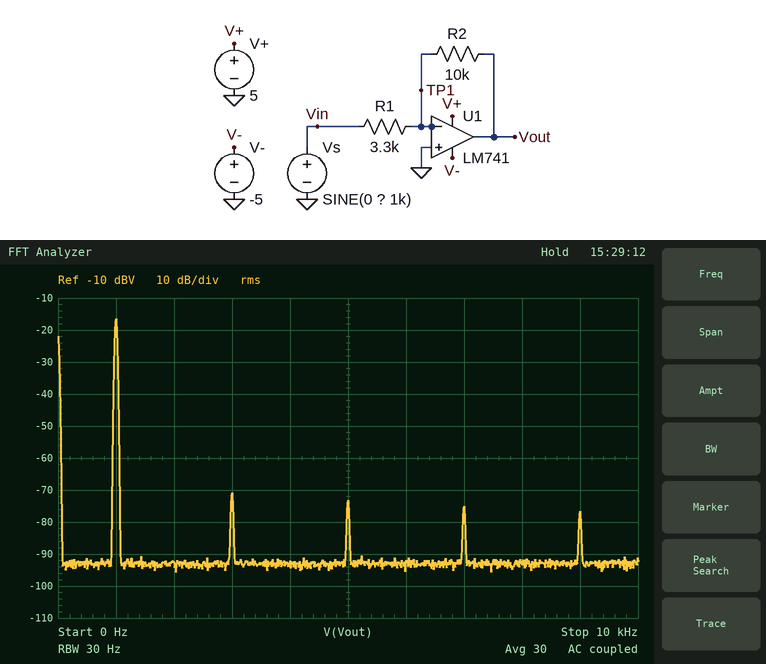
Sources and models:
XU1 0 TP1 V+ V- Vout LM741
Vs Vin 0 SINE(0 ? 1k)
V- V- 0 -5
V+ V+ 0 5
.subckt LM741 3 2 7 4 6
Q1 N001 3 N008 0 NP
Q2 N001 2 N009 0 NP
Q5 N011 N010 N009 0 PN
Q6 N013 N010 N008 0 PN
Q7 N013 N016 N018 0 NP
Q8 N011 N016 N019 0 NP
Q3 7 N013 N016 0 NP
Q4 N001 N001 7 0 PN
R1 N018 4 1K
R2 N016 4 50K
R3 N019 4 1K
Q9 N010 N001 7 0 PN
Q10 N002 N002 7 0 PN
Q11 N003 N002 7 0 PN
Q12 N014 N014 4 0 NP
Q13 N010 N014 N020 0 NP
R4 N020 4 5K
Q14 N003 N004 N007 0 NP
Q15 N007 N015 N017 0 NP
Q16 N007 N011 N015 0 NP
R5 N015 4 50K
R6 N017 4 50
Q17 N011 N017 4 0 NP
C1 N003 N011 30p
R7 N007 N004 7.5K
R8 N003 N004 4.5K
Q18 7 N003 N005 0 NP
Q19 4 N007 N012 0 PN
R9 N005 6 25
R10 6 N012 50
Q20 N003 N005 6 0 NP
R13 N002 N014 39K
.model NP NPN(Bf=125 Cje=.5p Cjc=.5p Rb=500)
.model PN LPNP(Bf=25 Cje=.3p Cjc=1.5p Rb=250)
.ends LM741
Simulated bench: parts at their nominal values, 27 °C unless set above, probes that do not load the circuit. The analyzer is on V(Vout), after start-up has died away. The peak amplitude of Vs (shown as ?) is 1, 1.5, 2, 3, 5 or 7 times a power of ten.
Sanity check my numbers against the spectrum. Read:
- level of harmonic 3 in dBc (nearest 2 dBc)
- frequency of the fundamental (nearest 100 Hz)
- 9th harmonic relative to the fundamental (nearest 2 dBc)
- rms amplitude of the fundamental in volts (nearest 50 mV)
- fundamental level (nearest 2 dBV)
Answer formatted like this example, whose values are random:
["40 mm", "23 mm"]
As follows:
["-54 dBc", "1.0 kHz", "-60 dBc", "150 mV", "-16 dBV"]
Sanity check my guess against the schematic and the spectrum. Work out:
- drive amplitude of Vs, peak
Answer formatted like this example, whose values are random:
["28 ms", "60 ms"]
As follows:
["70 mV"]
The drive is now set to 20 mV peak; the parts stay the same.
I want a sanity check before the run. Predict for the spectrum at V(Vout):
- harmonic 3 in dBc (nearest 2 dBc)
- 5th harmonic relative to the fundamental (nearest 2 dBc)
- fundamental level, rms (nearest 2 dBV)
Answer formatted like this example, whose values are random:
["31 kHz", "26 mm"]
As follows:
["-50 dBc", "-54 dBc", "-28 dBV"]
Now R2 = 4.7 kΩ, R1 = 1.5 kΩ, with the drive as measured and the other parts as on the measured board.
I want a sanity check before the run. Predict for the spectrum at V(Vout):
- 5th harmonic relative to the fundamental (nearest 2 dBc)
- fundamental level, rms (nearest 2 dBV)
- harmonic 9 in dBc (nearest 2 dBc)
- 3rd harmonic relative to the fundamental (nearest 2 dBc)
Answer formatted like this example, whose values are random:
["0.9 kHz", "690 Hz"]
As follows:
["-54 dBc", "-16 dBV", "-56 dBc", "-52 dBc"]
